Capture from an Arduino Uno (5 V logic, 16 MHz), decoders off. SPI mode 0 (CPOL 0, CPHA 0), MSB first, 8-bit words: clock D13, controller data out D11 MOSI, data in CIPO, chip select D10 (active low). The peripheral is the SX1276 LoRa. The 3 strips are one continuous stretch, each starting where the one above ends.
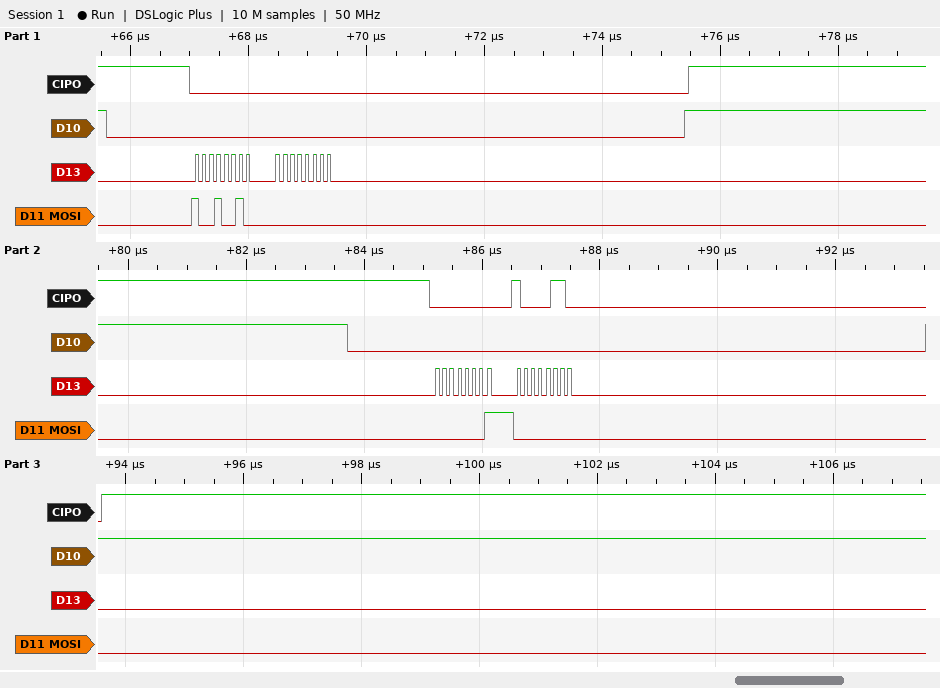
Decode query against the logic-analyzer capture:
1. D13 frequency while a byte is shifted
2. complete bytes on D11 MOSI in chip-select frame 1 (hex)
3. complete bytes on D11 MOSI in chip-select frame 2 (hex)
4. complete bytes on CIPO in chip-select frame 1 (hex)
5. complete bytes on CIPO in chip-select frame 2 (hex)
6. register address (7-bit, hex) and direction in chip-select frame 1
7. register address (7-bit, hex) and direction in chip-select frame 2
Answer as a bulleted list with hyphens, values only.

- 8 MHz
- 0x92 0x00
- 0x01 0x00
- 0x00 0x00
- 0x00 0x86
- 0x12 write
- 0x01 read
